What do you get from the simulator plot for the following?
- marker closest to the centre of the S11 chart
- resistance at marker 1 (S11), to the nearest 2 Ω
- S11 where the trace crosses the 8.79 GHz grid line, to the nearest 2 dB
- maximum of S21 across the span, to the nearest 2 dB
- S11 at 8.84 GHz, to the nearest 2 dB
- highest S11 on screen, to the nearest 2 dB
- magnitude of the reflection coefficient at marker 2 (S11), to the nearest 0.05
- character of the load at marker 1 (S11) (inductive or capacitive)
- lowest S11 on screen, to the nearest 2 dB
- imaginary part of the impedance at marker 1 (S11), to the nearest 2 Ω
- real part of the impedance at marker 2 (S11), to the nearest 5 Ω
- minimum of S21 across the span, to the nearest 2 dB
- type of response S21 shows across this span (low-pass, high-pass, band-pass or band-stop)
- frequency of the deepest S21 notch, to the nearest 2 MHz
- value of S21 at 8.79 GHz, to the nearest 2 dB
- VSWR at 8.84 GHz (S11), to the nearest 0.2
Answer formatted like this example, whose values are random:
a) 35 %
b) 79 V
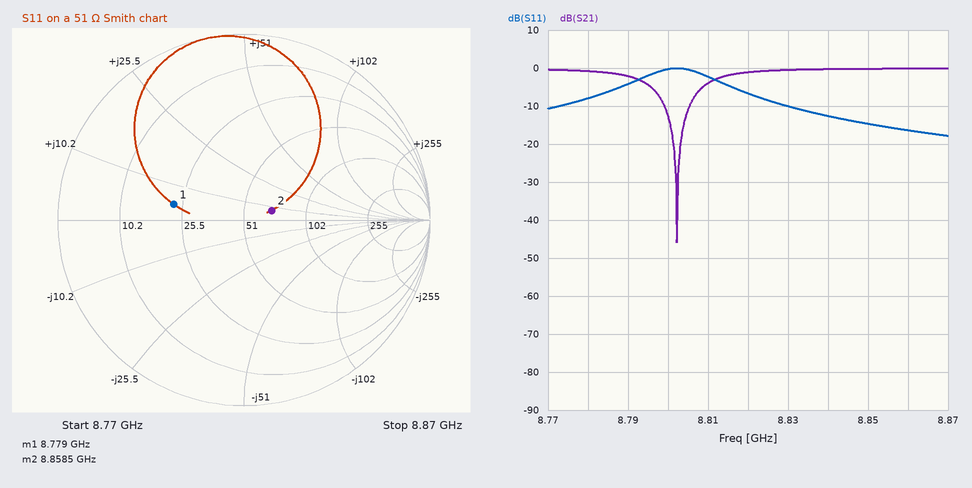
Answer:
a) marker 2
b) 22 Ω
c) -4 dB
d) 0 dB
e) -12 dB
f) 0 dB
g) 0.15
h) inductive
i) -18 dB
j) +4 Ω
k) 70 Ω
l) -46 dB
m) band-stop
n) 8.802 GHz
o) -2 dB
p) 1.6
